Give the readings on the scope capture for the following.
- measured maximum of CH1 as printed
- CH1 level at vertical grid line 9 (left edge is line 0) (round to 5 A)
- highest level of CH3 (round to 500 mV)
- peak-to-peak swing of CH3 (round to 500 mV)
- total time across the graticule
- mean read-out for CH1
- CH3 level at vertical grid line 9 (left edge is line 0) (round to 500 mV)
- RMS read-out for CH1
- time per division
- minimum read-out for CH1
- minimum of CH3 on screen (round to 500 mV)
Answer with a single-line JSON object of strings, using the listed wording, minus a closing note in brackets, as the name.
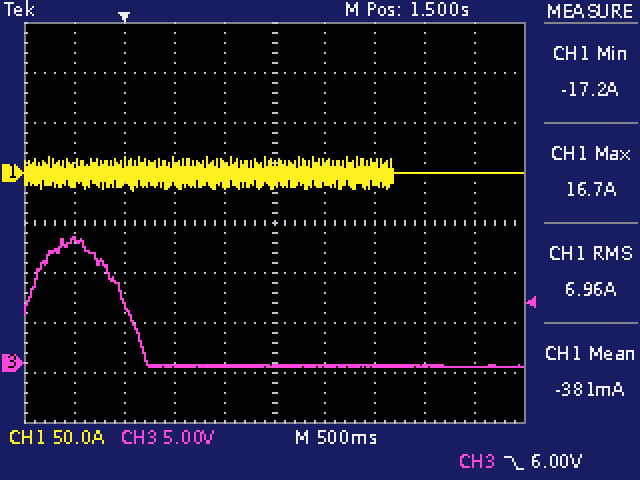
{"measured maximum of CH1 as printed": "16.7 A", "CH1 level at vertical grid line 9 (left edge is line 0)": "0 A", "highest level of CH3": "12.5 V", "peak-to-peak swing of CH3": "13.0 V", "total time across the graticule": "5 s", "mean read-out for CH1": "-381 mA", "CH3 level at vertical grid line 9 (left edge is line 0)": "-500 mV", "RMS read-out for CH1": "6.96 A", "time per division": "500 ms", "minimum read-out for CH1": "-17.2 A", "minimum of CH3 on screen": "-500 mV"}
